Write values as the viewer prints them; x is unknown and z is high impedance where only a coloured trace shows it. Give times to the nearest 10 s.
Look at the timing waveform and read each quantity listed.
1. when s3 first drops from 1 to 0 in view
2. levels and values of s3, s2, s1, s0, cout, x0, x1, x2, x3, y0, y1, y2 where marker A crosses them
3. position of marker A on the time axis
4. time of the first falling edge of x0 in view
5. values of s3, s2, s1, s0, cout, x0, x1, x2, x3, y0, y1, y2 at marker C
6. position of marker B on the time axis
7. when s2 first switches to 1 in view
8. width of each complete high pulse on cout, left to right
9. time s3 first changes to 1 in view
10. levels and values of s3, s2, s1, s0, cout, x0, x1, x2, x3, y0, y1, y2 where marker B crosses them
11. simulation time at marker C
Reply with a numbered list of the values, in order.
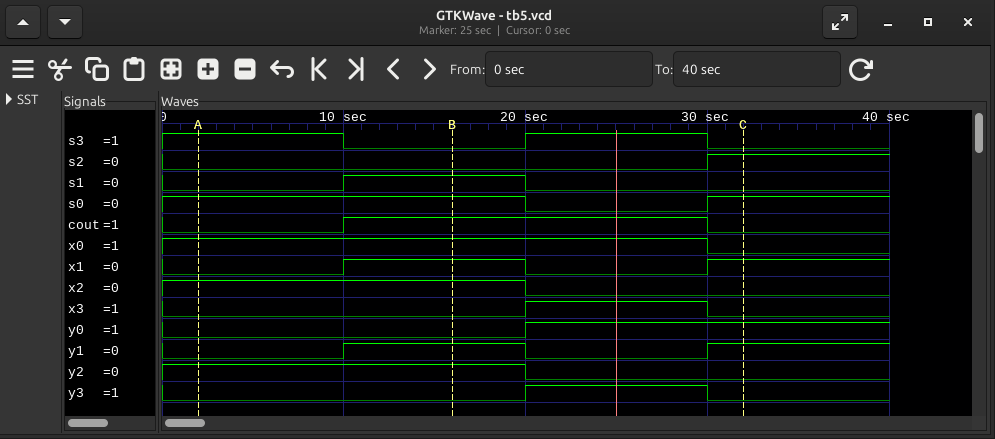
1. 10 s
2. s3=1, s2=0, s1=0, s0=1, cout=0, x0=1, x1=0, x2=1, x3=0, y0=0, y1=0, y2=1
3. 0 s
4. 30 s
5. s3=0, s2=1, s1=0, s0=1, cout=0, x0=0, x1=1, x2=0, x3=0, y0=1, y1=1, y2=0
6. 20 s
7. 30 s
8. 20 s
9. 20 s
10. s3=0, s2=0, s1=1, s0=1, cout=1, x0=1, x1=1, x2=1, x3=0, y0=0, y1=1, y2=1
11. 30 s
